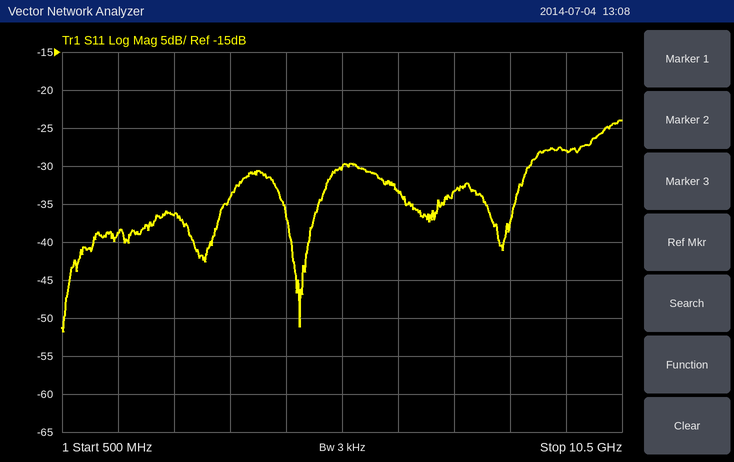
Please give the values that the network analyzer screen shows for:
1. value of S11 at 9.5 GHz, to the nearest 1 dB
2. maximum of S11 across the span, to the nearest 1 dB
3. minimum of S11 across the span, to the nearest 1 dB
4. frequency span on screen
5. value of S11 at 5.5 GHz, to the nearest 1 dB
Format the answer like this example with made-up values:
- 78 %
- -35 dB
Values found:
- -28 dB
- -24 dB
- -52 dB
- 10 GHz
- -30 dB
